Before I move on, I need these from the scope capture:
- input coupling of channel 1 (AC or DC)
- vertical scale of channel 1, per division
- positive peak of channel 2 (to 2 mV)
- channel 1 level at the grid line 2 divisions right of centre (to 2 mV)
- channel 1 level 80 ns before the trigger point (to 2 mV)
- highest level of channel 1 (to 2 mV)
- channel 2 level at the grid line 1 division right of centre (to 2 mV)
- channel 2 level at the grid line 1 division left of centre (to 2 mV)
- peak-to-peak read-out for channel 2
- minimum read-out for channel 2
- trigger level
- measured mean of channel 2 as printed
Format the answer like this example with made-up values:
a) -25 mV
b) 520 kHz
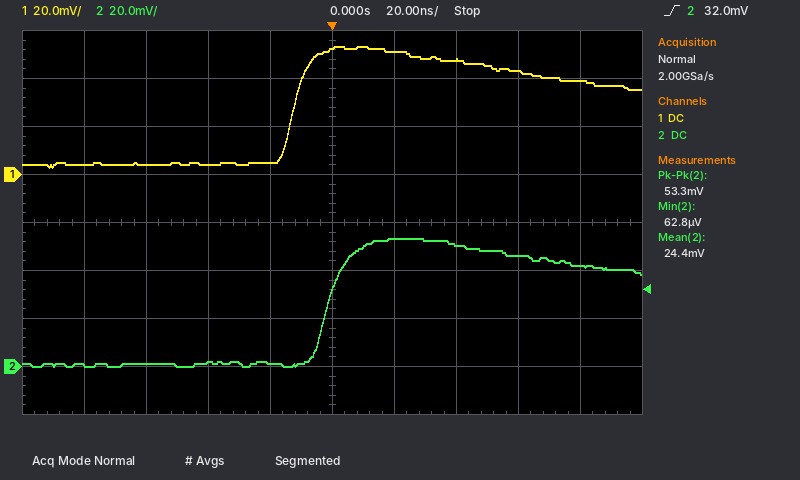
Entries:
a) DC
b) 20 mV
c) 54 mV
d) 48 mV
e) 4 mV
f) 54 mV
g) 54 mV
h) 2 mV
i) 53.3 mV
j) 62.8 µV
k) 32.0 mV
l) 24.4 mV
